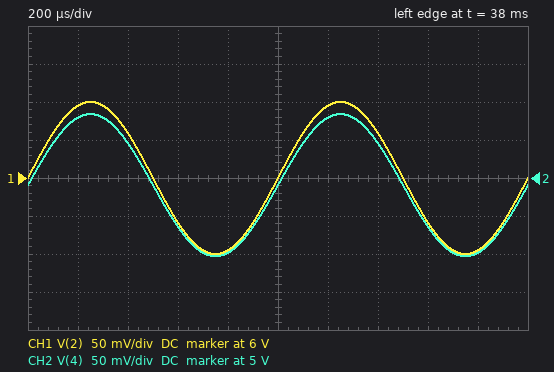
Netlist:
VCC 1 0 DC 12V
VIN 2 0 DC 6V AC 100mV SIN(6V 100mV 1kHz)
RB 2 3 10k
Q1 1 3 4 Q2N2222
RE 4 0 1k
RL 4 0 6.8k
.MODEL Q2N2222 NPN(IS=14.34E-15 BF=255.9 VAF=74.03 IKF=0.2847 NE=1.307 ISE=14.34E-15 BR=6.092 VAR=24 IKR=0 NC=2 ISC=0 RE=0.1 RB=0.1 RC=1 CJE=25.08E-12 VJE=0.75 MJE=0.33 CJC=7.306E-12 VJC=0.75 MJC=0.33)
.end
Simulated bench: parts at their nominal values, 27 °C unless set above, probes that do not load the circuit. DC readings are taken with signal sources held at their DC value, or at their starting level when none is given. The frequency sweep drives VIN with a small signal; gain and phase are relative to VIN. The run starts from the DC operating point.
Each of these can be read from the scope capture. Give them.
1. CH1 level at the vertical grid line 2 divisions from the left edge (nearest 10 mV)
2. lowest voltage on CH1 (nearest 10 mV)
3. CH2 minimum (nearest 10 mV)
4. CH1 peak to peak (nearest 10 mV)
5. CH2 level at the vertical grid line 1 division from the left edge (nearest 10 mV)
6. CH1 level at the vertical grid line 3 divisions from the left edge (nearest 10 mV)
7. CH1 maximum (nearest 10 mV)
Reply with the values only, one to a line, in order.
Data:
6.06 V
5.90 V
4.90 V
200 mV
5.08 V
5.94 V
6.10 V
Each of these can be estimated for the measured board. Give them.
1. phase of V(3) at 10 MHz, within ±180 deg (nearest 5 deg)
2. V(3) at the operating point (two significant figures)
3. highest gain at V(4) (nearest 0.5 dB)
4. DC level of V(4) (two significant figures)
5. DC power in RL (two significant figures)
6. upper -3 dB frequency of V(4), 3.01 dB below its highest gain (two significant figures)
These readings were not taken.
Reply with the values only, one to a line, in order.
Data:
-65 deg
5.7 V
-0.5 dB
5.0 V
3.7 mW
4.6 MHz
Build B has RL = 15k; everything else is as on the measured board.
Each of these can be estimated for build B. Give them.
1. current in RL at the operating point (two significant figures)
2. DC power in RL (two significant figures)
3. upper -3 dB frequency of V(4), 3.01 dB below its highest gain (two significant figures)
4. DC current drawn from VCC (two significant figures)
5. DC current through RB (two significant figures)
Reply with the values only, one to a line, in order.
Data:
330 µA
1.7 mW
4.5 MHz
5.3 mA
30 µA
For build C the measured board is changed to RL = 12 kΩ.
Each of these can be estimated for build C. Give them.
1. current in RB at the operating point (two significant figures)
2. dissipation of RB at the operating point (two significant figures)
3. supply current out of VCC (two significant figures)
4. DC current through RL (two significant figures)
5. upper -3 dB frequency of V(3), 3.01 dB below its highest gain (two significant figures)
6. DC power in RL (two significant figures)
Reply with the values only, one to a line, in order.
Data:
30 µA
9.2 µW
5.4 mA
420 µA
4.5 MHz
2.1 mW
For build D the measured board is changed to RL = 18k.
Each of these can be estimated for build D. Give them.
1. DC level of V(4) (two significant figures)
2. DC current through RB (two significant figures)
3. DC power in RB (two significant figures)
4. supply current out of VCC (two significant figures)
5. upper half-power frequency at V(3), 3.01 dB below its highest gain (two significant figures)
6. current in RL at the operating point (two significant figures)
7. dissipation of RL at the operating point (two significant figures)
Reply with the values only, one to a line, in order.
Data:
5.0 V
30 µA
8.8 µW
5.3 mA
4.5 MHz
280 µA
1.4 mW
